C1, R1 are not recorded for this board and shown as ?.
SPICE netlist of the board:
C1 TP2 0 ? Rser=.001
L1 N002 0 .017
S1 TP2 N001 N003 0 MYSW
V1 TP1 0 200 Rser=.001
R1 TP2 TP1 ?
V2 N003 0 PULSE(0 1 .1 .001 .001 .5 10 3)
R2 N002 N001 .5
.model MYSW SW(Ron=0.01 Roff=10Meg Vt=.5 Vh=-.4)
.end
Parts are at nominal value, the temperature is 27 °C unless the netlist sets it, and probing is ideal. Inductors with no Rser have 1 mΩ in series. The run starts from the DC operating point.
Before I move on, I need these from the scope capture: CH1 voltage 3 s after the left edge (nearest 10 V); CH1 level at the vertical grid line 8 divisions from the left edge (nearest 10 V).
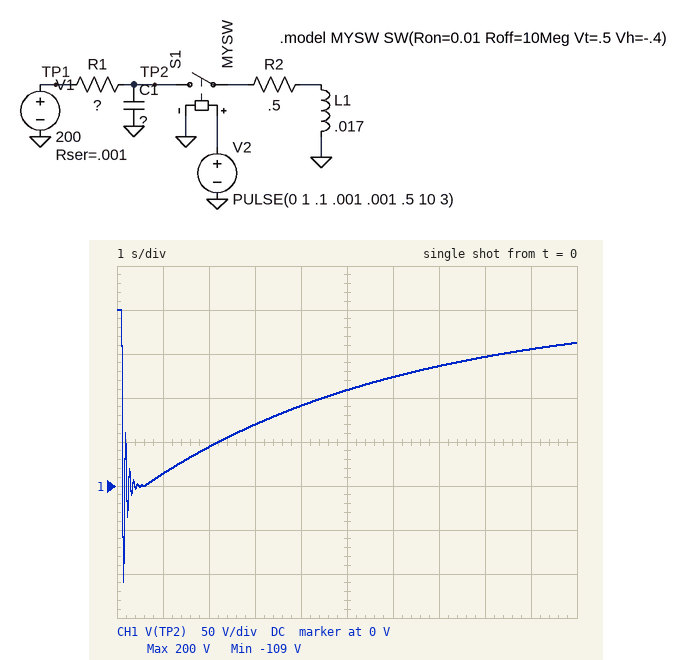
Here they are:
70 V
150 V
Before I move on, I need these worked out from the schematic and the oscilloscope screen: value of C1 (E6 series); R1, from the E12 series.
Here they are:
10 mF
560 Ω
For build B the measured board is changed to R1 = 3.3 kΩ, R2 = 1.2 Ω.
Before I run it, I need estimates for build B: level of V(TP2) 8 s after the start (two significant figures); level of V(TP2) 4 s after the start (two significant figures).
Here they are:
40 V
20 V
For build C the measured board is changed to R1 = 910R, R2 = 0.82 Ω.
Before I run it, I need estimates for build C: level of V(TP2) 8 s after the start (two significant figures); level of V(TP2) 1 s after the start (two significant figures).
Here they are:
110 V
8.7 V
